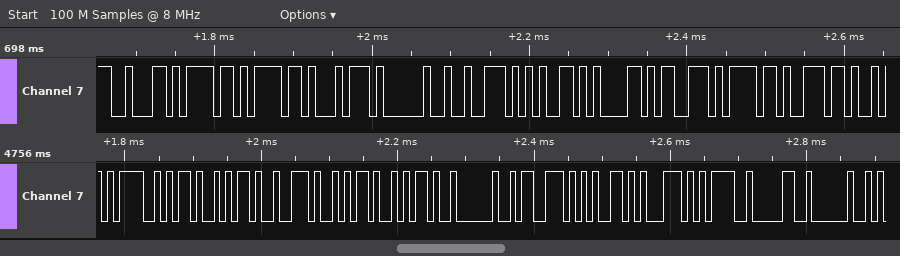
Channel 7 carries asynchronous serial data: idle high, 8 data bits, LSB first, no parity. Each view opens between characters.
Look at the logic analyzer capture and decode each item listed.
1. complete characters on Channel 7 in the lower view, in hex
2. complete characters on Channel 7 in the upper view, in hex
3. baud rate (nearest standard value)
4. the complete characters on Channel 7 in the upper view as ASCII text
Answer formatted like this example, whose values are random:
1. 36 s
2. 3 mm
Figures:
1. 3D, 2D, 2D, 2E, 2D, 2D, 20, 73, 65, 71, 3D, 30, 20
2. 62, 6F, 6F, 74, 20, 72, 65, 61, 73, 6F, 6E
3. 115200 baud
4. "boot reason"
